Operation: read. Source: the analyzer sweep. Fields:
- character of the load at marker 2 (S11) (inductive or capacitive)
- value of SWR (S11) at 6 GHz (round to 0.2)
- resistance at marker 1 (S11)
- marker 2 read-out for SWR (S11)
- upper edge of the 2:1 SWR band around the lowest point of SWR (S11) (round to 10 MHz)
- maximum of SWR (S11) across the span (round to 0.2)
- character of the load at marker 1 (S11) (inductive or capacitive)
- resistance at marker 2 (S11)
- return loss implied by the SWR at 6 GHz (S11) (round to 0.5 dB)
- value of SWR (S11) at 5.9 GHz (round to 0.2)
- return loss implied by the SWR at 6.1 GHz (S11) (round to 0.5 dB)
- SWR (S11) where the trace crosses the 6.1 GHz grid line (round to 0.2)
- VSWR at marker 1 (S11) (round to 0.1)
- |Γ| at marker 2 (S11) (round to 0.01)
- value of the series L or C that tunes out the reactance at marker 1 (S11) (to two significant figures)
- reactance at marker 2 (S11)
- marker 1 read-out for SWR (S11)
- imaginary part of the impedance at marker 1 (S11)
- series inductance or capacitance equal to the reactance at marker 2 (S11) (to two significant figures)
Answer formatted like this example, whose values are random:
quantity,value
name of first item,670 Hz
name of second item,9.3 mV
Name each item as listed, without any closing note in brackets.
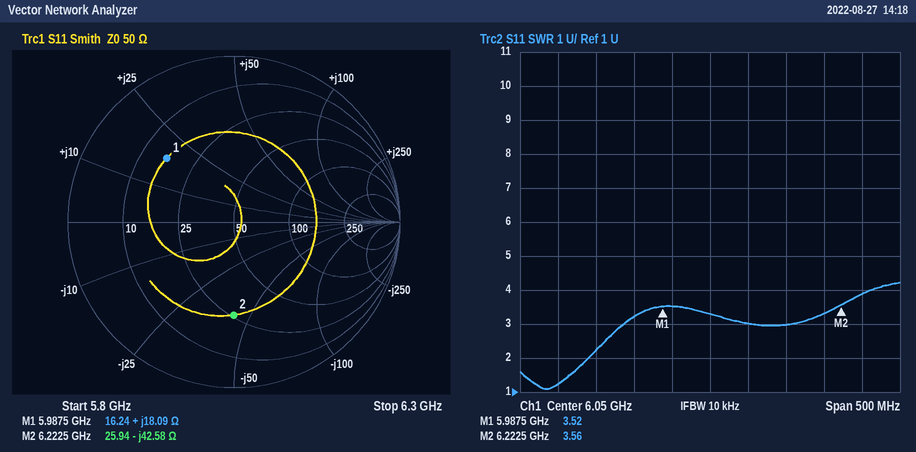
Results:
quantity,value
character of the load at marker 2 (S11),capacitive
value of SWR (S11) at 6 GHz,3.6
resistance at marker 1,16.24 Ω
marker 2 read-out for SWR,3.56
upper edge of the 2:1 SWR band around the lowest point of SWR (S11),5.89 GHz
maximum of SWR (S11) across the span,4.2
character of the load at marker 1 (S11),inductive
resistance at marker 2,25.94 Ω
return loss implied by the SWR at 6 GHz (S11),5.0 dB
value of SWR (S11) at 5.9 GHz,2.2
return loss implied by the SWR at 6.1 GHz (S11),6.0 dB
SWR (S11) where the trace crosses the 6.1 GHz grid line,3.0
VSWR at marker 1 (S11),3.5
|Γ| at marker 2 (S11),0.56
value of the series L or C that tunes out the reactance at marker 1 (S11),1.5 pF
reactance at marker 2,-42.58 Ω
marker 1 read-out for SWR,3.52
imaginary part of the impedance at marker 1,+18.09 Ω
series inductance or capacitance equal to the reactance at marker 2 (S11),600 fF
